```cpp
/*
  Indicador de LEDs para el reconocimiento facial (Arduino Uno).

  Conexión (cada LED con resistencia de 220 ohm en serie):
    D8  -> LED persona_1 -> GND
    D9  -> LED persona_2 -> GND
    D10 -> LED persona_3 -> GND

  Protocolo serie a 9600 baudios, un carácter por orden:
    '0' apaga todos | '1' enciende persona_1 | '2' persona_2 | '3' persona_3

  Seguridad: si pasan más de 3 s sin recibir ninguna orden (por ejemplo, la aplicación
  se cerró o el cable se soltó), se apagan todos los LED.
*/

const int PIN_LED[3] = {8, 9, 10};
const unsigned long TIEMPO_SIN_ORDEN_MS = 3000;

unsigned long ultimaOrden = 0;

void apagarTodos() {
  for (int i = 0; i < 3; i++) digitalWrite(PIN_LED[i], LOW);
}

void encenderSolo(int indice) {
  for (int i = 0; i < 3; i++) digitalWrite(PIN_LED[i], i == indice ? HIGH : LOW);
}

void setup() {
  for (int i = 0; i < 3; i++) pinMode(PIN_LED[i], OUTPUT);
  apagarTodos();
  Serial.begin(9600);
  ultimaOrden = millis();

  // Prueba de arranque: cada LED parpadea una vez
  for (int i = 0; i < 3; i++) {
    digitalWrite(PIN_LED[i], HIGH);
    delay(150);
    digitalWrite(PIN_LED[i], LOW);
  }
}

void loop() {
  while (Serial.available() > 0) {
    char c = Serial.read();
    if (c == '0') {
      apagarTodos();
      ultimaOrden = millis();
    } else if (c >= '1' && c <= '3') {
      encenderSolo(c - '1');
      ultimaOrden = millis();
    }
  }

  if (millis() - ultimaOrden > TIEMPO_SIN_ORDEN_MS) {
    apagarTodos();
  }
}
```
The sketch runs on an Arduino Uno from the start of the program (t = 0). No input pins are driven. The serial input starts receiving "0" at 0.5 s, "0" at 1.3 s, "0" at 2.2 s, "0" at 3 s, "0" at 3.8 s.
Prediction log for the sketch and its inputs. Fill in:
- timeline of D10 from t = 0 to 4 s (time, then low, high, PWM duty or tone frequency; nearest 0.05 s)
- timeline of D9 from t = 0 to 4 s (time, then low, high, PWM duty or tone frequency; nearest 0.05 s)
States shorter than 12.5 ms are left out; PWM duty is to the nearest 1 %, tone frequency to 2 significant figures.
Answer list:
0 s low; 0.3 s high; 0.45 s low
0 s low; 0.15 s high; 0.3 s low
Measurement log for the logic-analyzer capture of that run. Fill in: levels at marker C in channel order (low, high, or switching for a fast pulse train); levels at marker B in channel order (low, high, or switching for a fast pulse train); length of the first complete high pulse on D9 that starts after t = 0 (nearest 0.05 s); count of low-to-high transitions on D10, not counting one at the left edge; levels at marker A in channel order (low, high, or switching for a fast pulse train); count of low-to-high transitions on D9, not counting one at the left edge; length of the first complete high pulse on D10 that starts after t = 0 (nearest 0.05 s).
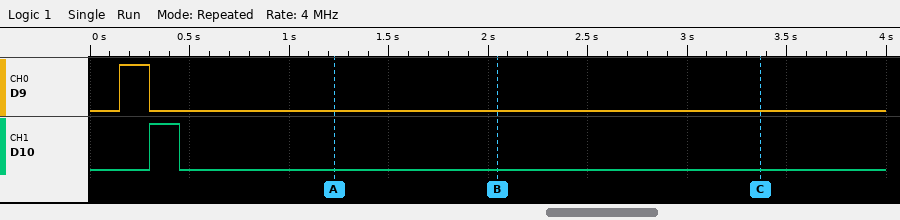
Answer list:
D9 low, D10 low
D9 low, D10 low
0.15 s
1
D9 low, D10 low
1
0.15 s
